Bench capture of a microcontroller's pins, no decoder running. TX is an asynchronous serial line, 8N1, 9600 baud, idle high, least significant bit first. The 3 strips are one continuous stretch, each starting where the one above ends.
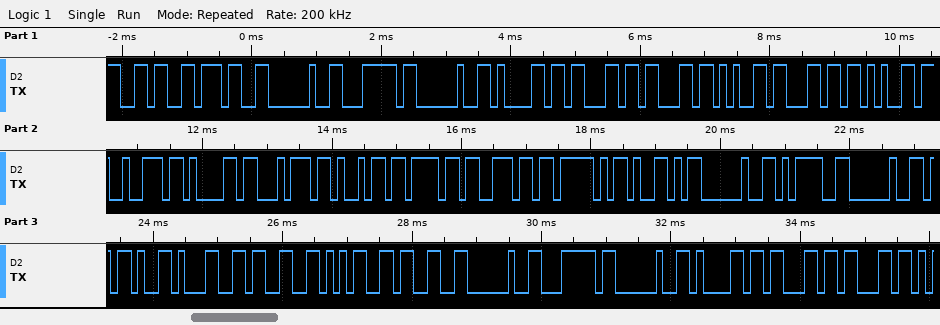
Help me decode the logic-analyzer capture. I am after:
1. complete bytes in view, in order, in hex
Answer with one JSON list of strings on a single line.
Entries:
["0x36 0x37 0x20 0x7C 0x20 0x61 0x63 0x63 0x65 0x6C 0x65 0x72 0x61 0x74 0x69 0x6F 0x6E 0x5F 0x59 0x20 0x3D 0x20 0x2D 0x31 0x33 0x35 0x33 0x20 0x7C 0x20 0x61 0x63 0x63"]
